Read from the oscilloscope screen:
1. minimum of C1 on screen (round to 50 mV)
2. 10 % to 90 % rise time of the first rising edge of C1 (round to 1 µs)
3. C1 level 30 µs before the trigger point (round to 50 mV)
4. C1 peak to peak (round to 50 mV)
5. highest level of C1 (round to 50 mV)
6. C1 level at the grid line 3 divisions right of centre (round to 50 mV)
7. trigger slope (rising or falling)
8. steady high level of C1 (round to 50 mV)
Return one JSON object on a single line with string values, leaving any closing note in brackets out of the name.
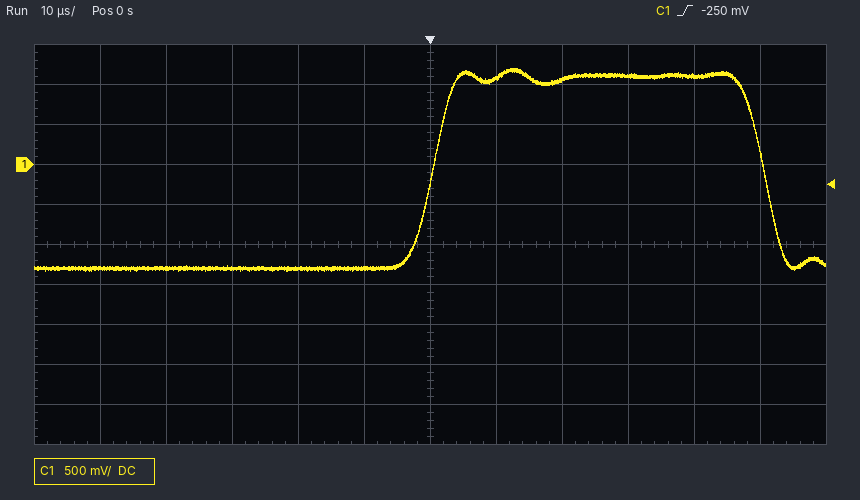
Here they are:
{"minimum of C1 on screen": "-1.35 V", "10 % to 90 % rise time of the first rising edge of C1": "6 µs", "C1 level 30 µs before the trigger point": "-1.30 V", "C1 peak to peak": "2.55 V", "highest level of C1": "1.20 V", "C1 level at the grid line 3 divisions right of centre": "1.10 V", "trigger slope": "rising", "steady high level of C1": "1.10 V"}
